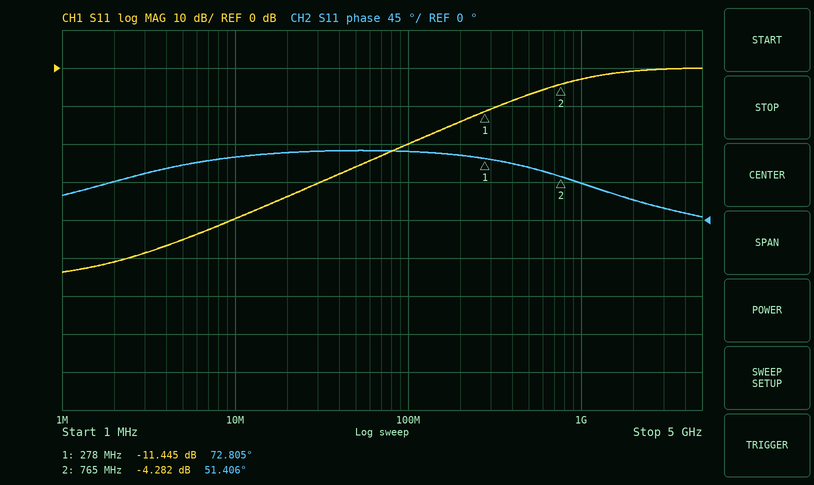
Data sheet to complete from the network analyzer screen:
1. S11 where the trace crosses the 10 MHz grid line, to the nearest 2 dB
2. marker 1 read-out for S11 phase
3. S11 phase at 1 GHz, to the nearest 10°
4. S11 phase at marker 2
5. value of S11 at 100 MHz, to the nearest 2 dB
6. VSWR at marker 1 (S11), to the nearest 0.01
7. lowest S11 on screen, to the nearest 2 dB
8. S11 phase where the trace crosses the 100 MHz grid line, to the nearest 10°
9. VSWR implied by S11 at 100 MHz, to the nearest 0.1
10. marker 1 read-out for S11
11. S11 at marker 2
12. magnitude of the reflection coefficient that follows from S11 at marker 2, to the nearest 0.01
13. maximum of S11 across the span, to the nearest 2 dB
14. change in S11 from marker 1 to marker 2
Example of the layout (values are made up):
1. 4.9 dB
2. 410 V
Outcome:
1. -40 dB
2. 72.805°
3. 40°
4. 51.406°
5. -20 dB
6. 1.73
7. -54 dB
8. 80°
9. 1.2
10. -11.445 dB
11. -4.282 dB
12. 0.61
13. 0 dB
14. 7.163 dB
